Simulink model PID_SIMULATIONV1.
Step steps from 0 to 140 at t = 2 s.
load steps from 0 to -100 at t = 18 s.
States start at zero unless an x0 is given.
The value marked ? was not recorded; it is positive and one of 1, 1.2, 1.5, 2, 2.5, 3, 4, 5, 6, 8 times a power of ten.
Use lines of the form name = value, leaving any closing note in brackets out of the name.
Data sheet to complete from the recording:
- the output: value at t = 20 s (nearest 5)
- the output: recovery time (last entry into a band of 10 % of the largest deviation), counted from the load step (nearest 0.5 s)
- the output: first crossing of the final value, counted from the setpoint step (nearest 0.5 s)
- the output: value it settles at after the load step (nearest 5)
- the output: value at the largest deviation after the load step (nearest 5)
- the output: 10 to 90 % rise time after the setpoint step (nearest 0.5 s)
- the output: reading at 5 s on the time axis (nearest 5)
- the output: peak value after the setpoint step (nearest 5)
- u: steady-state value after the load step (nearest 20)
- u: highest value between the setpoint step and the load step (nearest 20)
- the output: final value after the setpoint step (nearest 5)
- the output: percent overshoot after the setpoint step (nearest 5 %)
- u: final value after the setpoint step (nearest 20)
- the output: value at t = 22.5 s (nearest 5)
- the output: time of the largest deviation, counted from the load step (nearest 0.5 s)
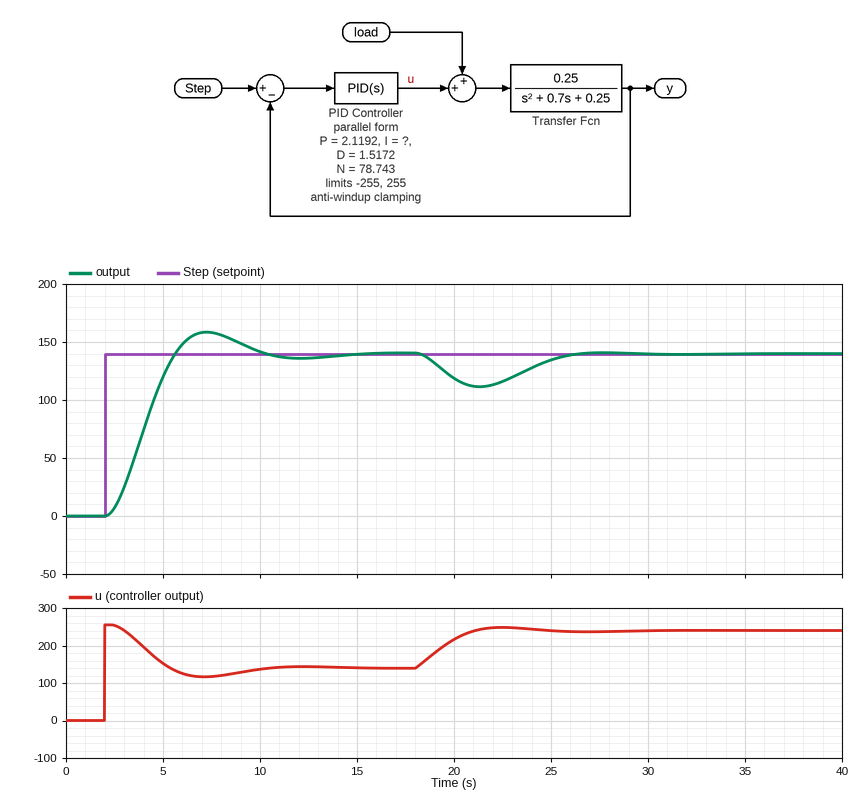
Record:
the output: value at t = 20 s = 120
the output: recovery time (last entry into a band of 10 % of the largest deviation), counted from the load step = 7.5 s
the output: first crossing of the final value, counted from the setpoint step = 3.5 s
the output: value it settles at after the load step = 140
the output: value at the largest deviation after the load step = 110
the output: 10 to 90 % rise time after the setpoint step = 2.5 s
the output: reading at 5 s on the time axis = 120
the output: peak value after the setpoint step = 160
u: steady-state value after the load step = 240
u: highest value between the setpoint step and the load step = 260
the output: final value after the setpoint step = 140
the output: percent overshoot after the setpoint step = 15 %
u: final value after the setpoint step = 140
the output: value at t = 22.5 s = 115
the output: time of the largest deviation, counted from the load step = 3.5 s
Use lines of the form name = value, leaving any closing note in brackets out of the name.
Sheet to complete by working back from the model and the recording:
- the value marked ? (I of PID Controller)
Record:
the value marked ? = 0.8
